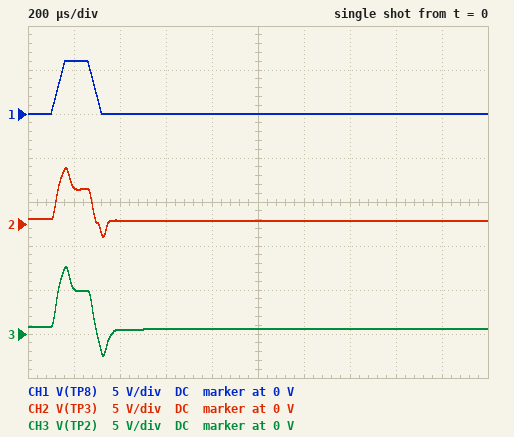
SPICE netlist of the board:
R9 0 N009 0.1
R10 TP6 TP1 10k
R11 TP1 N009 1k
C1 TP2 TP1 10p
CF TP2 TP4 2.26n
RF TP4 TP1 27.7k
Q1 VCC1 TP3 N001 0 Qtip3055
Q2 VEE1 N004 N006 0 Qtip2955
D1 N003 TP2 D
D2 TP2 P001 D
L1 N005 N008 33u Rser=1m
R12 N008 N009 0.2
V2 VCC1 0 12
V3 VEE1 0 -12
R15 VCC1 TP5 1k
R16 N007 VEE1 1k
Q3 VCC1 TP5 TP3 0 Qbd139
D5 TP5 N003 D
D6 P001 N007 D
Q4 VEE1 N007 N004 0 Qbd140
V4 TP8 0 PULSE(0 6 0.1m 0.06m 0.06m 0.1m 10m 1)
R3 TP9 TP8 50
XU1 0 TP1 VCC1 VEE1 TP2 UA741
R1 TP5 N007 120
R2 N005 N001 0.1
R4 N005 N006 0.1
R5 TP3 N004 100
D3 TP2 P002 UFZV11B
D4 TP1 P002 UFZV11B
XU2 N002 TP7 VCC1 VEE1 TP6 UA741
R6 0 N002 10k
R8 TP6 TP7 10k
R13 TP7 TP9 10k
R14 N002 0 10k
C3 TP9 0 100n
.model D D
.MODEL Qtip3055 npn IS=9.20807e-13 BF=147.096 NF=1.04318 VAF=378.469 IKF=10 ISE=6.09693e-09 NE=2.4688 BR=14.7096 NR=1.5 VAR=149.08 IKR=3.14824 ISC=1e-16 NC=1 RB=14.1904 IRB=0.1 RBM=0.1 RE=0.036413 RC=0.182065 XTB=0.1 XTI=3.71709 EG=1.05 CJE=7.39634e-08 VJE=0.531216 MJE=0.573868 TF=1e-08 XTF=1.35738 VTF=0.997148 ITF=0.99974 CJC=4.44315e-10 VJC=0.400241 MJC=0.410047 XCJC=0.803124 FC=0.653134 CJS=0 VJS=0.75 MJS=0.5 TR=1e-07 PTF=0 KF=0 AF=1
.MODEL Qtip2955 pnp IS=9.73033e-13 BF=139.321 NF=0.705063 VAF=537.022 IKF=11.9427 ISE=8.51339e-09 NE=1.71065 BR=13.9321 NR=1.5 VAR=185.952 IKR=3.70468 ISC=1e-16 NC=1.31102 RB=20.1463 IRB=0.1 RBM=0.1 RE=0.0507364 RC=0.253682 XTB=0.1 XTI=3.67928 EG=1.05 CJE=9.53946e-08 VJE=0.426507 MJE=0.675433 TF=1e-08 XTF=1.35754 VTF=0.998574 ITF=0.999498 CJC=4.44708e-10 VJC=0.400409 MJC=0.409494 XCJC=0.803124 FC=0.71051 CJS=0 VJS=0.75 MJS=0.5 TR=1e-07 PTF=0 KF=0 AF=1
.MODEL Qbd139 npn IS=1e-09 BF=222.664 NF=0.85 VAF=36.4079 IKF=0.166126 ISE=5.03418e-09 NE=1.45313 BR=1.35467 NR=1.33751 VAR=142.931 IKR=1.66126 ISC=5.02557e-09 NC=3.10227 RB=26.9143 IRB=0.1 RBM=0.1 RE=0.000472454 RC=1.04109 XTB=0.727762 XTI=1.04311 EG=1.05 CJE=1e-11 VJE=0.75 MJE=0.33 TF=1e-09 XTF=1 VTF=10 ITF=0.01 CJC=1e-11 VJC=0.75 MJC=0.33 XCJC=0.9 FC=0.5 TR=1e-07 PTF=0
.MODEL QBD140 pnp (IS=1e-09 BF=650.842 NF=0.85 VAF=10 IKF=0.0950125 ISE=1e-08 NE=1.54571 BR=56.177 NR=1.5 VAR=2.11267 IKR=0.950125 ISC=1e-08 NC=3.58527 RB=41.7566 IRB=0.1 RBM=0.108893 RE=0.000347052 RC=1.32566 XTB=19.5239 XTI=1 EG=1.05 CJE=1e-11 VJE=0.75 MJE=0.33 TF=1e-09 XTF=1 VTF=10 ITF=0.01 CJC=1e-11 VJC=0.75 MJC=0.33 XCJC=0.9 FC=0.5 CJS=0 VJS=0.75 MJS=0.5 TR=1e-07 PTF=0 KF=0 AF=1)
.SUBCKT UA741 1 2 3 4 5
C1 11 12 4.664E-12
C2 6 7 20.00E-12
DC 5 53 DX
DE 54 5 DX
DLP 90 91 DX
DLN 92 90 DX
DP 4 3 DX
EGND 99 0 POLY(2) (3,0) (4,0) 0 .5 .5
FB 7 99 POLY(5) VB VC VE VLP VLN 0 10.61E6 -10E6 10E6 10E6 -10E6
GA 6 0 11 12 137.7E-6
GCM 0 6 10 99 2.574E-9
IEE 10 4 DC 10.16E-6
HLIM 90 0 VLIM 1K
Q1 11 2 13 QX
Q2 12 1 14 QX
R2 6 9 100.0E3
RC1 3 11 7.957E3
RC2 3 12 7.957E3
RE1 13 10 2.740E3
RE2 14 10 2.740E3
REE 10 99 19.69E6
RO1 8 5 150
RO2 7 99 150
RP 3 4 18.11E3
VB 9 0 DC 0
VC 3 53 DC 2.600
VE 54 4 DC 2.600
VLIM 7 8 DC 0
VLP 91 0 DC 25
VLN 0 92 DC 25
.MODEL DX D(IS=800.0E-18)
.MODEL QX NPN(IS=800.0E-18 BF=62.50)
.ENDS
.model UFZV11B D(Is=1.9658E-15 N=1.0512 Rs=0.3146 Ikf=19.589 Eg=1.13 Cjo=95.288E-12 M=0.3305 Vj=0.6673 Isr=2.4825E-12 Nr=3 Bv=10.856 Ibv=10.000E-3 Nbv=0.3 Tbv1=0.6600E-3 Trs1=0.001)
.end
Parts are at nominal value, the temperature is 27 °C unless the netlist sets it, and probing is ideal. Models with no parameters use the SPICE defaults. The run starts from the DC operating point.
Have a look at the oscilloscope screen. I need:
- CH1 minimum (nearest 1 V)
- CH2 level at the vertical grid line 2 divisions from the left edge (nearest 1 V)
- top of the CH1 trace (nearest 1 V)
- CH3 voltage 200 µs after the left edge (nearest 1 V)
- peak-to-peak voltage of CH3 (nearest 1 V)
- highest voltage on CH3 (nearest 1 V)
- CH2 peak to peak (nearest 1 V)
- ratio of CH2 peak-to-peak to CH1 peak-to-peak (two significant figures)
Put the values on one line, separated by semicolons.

0 V; 0 V; 6 V; 5 V; 10 V; 8 V; 8 V; 1.3
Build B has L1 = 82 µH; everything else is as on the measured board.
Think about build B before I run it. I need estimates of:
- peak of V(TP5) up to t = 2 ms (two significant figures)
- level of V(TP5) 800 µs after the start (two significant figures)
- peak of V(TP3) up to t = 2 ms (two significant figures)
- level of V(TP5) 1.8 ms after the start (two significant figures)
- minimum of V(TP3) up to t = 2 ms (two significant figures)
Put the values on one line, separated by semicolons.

8.9 V; 610 mV; 8.5 V; 650 mV; -6.0 V
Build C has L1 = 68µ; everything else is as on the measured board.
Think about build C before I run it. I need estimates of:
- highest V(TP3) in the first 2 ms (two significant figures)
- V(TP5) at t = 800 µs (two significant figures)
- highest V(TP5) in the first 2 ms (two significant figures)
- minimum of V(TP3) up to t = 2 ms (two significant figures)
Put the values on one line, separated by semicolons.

8.5 V; 610 mV; 8.9 V; -4.9 V
